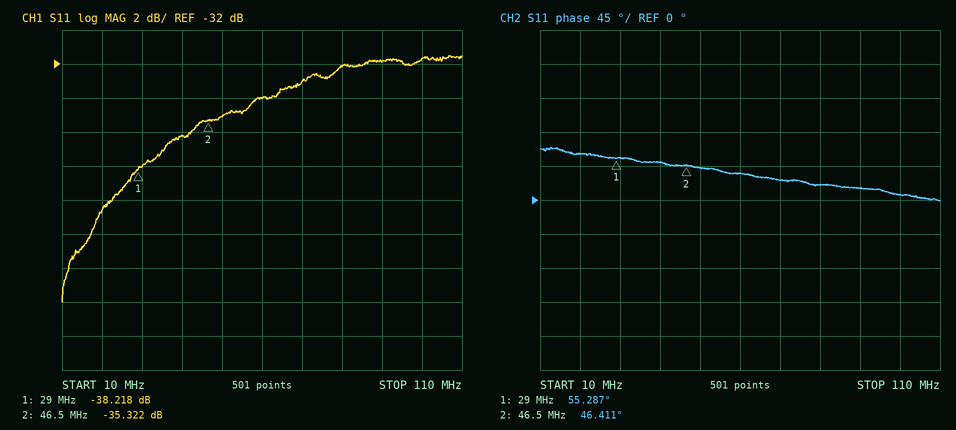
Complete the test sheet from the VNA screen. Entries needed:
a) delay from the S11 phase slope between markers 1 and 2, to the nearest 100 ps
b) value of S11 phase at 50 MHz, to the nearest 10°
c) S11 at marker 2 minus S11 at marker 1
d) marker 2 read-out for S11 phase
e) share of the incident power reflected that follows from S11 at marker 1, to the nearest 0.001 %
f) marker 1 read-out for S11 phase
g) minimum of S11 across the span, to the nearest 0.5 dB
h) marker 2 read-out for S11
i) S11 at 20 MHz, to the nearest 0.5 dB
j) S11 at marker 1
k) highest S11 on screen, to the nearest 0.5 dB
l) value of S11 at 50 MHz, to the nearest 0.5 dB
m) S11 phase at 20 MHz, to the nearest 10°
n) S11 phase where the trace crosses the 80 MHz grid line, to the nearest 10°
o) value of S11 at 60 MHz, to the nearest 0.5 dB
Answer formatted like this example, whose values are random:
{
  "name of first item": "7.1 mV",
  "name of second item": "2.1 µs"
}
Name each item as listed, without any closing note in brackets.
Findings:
{
  "delay from the S11 phase slope between markers 1 and 2, to the nearest 100 ps": "1.4 ns",
  "value of S11 phase at 50 MHz, to the nearest 10°": "40°",
  "S11 at marker 2 minus S11 at marker 1": "2.896 dB",
  "marker 2 read-out for S11 phase": "46.411°",
  "share of the incident power reflected that follows from S11 at marker 1, to the nearest 0.001 %": "0.015 %",
  "marker 1 read-out for S11 phase": "55.287°",
  "minimum of S11 across the span, to the nearest 0.5 dB": "-46.0 dB",
  "marker 2 read-out for S11": "-35.322 dB",
  "S11 at 20 MHz, to the nearest 0.5 dB": "-40.5 dB",
  "S11 at marker 1": "-38.218 dB",
  "highest S11 on screen, to the nearest 0.5 dB": "-31.5 dB",
  "value of S11 at 50 MHz, to the nearest 0.5 dB": "-35.0 dB",
  "S11 phase at 20 MHz, to the nearest 10°": "60°",
  "S11 phase where the trace crosses the 80 MHz grid line, to the nearest 10°": "20°",
  "value of S11 at 60 MHz, to the nearest 0.5 dB": "-34.0 dB"
}
